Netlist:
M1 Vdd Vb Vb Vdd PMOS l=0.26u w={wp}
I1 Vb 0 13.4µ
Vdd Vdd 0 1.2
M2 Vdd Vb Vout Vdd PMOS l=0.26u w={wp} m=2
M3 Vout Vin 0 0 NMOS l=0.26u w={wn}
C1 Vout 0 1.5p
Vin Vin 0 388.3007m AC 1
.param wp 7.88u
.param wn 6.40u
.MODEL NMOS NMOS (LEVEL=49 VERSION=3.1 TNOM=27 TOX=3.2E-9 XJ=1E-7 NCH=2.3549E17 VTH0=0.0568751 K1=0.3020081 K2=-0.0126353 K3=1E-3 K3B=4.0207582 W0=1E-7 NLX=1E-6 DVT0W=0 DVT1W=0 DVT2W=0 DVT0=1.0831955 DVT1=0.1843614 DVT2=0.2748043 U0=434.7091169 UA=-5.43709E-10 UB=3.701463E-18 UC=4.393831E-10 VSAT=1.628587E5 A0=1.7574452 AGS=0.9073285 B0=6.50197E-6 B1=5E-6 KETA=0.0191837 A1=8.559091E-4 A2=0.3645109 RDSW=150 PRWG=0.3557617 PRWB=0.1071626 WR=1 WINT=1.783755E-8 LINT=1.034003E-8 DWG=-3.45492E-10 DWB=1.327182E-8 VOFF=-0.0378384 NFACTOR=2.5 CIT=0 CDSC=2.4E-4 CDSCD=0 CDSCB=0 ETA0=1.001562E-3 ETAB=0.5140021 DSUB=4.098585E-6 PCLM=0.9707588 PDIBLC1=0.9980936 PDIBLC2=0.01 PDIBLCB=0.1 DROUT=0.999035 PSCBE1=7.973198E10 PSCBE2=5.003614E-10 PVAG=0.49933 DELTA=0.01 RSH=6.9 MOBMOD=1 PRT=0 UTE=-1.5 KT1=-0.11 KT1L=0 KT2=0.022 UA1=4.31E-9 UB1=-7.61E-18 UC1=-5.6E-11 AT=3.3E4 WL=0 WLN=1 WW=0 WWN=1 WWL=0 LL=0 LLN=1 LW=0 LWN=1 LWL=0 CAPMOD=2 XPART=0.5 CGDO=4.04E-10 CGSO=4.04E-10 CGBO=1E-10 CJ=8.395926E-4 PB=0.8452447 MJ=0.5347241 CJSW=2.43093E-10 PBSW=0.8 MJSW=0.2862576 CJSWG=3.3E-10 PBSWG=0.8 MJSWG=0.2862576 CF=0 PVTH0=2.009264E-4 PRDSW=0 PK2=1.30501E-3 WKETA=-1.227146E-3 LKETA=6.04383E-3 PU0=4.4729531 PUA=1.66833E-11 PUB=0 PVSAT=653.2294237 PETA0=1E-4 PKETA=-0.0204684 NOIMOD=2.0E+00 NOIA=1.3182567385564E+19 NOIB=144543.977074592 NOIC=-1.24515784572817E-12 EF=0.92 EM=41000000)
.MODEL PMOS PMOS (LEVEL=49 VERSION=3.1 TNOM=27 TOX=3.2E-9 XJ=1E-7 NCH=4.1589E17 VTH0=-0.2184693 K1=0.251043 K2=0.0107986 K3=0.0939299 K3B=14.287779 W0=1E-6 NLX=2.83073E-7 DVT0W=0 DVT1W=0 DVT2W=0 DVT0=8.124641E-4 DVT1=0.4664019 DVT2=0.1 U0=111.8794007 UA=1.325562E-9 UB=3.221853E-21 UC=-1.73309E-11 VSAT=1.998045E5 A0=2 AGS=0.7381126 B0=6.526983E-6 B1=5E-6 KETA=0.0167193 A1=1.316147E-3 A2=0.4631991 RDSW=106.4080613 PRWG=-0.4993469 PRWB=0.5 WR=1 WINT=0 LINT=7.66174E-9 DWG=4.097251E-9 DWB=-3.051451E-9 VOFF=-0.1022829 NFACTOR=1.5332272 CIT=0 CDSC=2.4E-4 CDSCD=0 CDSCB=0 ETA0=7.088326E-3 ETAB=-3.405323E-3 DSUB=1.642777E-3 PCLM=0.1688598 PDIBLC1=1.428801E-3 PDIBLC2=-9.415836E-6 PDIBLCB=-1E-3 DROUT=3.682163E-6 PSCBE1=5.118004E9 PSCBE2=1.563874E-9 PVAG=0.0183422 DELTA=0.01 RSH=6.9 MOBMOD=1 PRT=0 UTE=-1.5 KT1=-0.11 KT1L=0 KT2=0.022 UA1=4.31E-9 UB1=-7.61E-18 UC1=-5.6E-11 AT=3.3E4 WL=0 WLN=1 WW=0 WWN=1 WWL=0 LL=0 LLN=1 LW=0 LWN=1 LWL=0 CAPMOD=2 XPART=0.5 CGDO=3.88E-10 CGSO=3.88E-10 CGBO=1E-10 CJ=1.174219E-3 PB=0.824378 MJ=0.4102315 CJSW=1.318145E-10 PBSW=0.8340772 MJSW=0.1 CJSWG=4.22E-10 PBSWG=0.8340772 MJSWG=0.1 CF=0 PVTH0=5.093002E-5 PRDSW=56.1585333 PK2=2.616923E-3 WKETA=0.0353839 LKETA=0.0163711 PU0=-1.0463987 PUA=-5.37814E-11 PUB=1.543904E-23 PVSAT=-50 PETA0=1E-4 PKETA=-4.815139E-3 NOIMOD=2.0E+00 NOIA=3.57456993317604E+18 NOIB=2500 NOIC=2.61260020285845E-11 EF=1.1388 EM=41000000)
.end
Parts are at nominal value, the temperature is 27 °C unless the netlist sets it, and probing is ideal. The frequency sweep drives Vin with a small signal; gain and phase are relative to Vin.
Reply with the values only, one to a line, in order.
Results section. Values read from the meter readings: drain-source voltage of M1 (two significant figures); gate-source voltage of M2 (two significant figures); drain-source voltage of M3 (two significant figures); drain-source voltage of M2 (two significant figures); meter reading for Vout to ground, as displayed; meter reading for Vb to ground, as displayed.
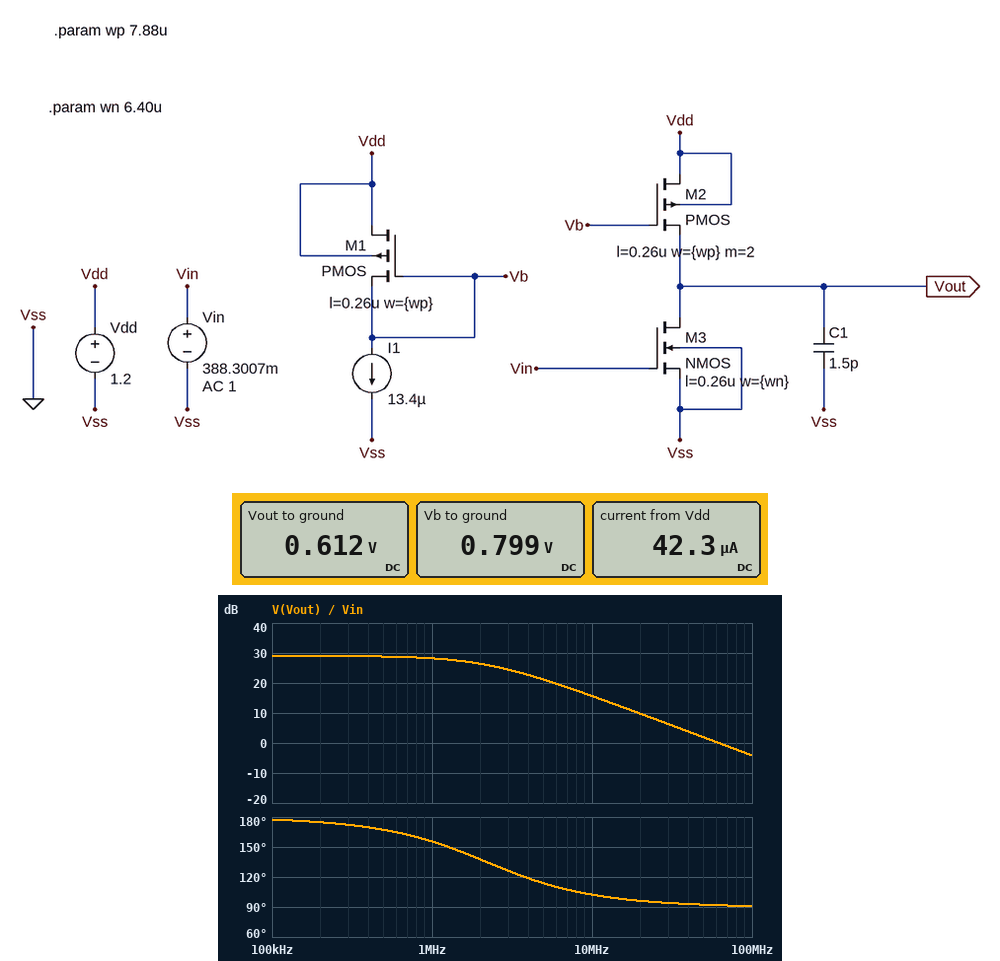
400 mV
190 mV
610 mV
590 mV
0.612 V
0.799 V
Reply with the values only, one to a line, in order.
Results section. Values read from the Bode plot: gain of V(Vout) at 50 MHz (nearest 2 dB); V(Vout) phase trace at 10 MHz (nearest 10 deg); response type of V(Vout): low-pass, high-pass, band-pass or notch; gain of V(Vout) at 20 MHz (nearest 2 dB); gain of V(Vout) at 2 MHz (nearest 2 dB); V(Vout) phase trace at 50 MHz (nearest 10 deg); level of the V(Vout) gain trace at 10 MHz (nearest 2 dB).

2 dB
100 deg
low-pass
10 dB
26 dB
90 deg
16 dB
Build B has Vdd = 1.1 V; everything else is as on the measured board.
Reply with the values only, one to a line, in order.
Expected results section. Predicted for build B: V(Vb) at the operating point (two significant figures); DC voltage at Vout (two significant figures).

700 mV
560 mV
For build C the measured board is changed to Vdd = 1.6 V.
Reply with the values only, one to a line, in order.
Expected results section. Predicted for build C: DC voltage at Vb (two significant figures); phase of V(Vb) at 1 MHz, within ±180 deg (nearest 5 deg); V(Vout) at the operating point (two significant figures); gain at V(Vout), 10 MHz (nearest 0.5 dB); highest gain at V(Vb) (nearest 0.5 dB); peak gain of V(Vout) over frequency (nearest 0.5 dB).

1.2 V
-115 deg
840 mV
16.0 dB
-40.0 dB
29.5 dB
